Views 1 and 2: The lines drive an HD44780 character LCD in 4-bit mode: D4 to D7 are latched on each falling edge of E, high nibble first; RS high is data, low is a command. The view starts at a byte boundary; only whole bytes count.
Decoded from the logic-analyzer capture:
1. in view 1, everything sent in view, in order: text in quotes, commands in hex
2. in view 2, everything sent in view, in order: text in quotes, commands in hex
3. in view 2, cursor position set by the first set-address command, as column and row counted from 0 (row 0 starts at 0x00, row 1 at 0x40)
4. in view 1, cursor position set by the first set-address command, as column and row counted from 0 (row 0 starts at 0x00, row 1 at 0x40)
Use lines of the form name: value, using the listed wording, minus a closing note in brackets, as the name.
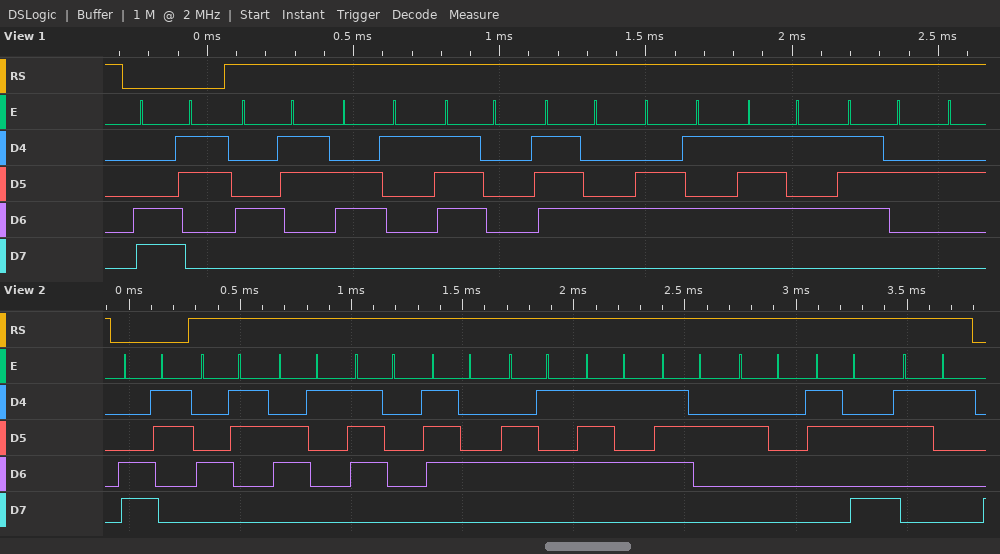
in view 1, everything sent in view, in order: text in quotes, commands in hex: 0xC3 "Capteur"
in view 2, everything sent in view, in order: text in quotes, commands in hex: 0xC3 "Capteur :1"
in view 2, cursor position set by the first set-address command, as column and row counted from 0: column 3, row 1
in view 1, cursor position set by the first set-address command, as column and row counted from 0: column 3, row 1
